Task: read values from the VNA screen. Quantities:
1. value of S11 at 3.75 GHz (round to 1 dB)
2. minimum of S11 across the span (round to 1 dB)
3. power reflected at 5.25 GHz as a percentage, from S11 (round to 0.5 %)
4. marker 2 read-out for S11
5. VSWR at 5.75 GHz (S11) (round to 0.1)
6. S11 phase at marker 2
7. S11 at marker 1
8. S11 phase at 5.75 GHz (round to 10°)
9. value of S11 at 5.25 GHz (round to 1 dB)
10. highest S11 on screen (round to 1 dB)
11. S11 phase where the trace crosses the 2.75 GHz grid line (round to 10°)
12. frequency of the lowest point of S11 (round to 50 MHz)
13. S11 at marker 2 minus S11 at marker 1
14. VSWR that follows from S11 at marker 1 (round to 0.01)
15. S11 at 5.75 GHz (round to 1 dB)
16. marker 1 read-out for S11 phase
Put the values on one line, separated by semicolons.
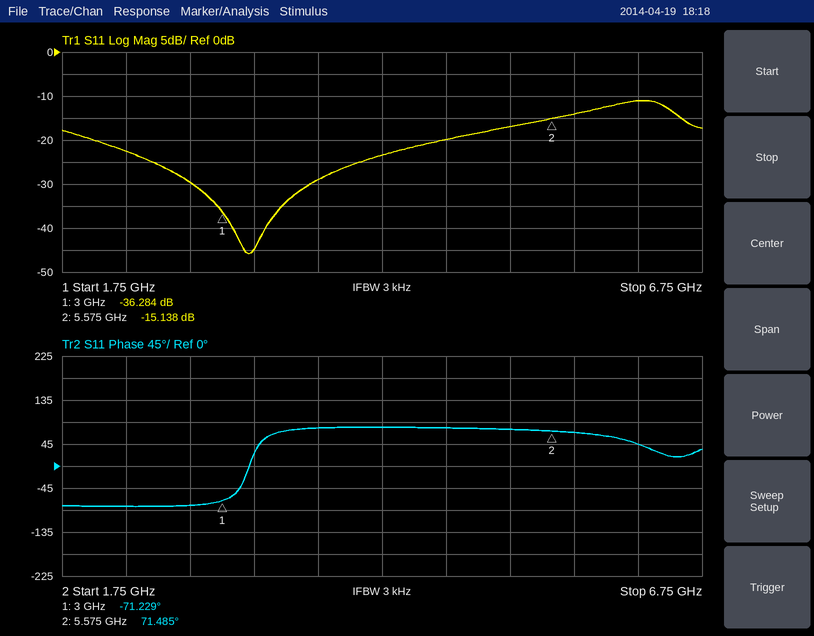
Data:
-29 dB; -46 dB; 2.0 %; -15.138 dB; 1.5; 71.485°; -36.284 dB; 70°; -17 dB; -11 dB; -80°; 3.20 GHz; 21.146 dB; 1.03; -14 dB; -71.229°
